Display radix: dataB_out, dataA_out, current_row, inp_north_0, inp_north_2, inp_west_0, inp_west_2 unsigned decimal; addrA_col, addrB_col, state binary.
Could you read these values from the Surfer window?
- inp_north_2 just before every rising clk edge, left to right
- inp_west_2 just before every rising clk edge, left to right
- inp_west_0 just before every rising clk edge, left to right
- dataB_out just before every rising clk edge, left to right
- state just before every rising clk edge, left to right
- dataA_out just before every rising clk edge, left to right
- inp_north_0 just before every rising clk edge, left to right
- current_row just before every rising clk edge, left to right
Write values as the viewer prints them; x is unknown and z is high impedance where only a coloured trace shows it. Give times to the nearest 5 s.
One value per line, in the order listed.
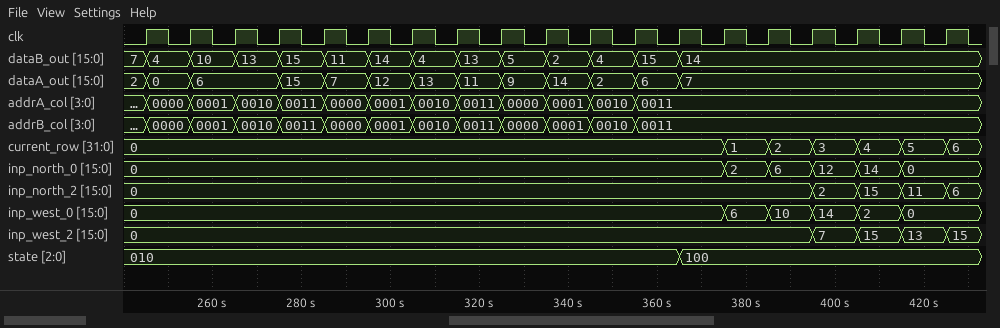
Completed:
0, 0, 0, 0, 0, 0, 0, 0, 0, 0, 0, 0, 0, 0, 0, 0, 2, 15, 11
0, 0, 0, 0, 0, 0, 0, 0, 0, 0, 0, 0, 0, 0, 0, 0, 7, 15, 13
0, 0, 0, 0, 0, 0, 0, 0, 0, 0, 0, 0, 0, 0, 6, 10, 14, 2, 0
7, 4, 10, 13, 15, 11, 14, 4, 13, 5, 2, 4, 15, 14, 14, 14, 14, 14, 14
010, 010, 010, 010, 010, 010, 010, 010, 010, 010, 010, 010, 010, 100, 100, 100, 100, 100, 100
2, 0, 6, 6, 15, 7, 12, 13, 11, 9, 14, 2, 6, 7, 7, 7, 7, 7, 7
0, 0, 0, 0, 0, 0, 0, 0, 0, 0, 0, 0, 0, 0, 2, 6, 12, 14, 0
0, 0, 0, 0, 0, 0, 0, 0, 0, 0, 0, 0, 0, 0, 1, 2, 3, 4, 5
